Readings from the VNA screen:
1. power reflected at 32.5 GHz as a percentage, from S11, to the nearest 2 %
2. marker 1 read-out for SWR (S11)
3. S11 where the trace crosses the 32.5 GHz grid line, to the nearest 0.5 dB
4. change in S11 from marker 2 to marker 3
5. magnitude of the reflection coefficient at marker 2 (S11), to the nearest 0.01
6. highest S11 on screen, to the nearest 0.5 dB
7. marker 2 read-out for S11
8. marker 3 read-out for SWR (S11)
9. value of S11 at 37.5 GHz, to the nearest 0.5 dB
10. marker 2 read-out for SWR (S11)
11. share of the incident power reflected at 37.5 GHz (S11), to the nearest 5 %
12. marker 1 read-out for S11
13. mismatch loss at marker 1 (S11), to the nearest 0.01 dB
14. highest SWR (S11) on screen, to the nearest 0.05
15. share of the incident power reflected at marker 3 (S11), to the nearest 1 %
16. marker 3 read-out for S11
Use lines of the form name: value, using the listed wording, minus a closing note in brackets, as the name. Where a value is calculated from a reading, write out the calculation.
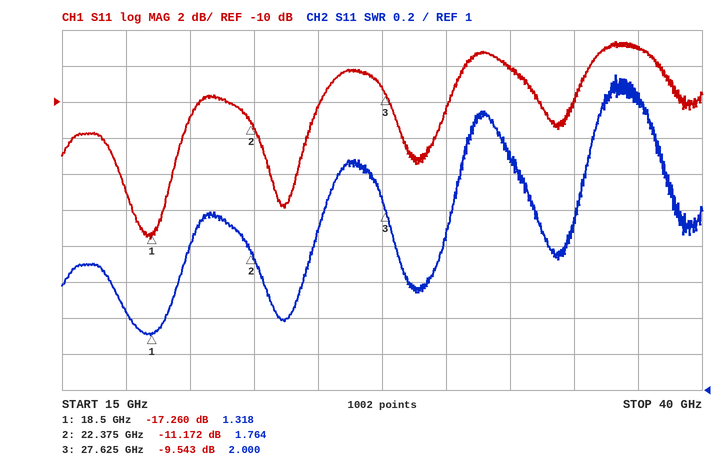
power reflected at 32.5 GHz as a percentage, from S11, to the nearest 2 %: 10^(-8/10) ≈ 16 %
marker 1 read-out for SWR: 1.318
S11 where the trace crosses the 32.5 GHz grid line, to the nearest 0.5 dB: -8.0 dB
change in S11 from marker 2 to marker 3: -9.543 − (-11.172) = 1.629 dB
magnitude of the reflection coefficient at marker 2 (S11), to the nearest 0.01: 10^(-11.172/20) ≈ 0.28
highest S11 on screen, to the nearest 0.5 dB: -6.5 dB
marker 2 read-out for S11: -11.172 dB
marker 3 read-out for SWR: 2.000
value of S11 at 37.5 GHz, to the nearest 0.5 dB: -7.0 dB
marker 2 read-out for SWR: 1.764
share of the incident power reflected at 37.5 GHz (S11), to the nearest 5 %: 10^(-7/10) ≈ 20 %
marker 1 read-out for S11: -17.260 dB
mismatch loss at marker 1 (S11), to the nearest 0.01 dB: −10 log10(1 − 10^(-17.26/10)) ≈ 0.08 dB
highest SWR (S11) on screen, to the nearest 0.05: 2.75
share of the incident power reflected at marker 3 (S11), to the nearest 1 %: 10^(-9.543/10) ≈ 11 %
marker 3 read-out for S11: -9.543 dB
